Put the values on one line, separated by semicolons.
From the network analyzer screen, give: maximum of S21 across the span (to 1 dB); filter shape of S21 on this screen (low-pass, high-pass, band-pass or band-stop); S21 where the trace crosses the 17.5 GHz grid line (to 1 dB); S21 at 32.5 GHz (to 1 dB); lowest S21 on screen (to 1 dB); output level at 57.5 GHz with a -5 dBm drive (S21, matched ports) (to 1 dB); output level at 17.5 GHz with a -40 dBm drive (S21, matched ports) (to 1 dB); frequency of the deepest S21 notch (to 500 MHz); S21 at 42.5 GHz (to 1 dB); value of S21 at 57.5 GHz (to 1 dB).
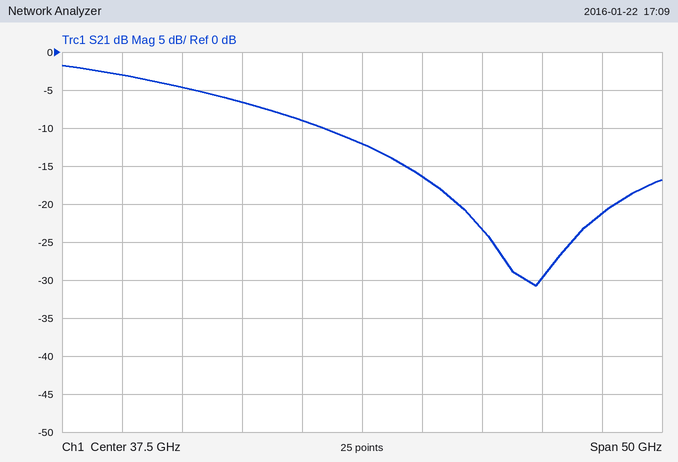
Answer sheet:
-2 dB; low-pass; -3 dB; -9 dB; -31 dB; -26 dBm; -43 dBm; 52.0 GHz; -16 dB; -21 dB
